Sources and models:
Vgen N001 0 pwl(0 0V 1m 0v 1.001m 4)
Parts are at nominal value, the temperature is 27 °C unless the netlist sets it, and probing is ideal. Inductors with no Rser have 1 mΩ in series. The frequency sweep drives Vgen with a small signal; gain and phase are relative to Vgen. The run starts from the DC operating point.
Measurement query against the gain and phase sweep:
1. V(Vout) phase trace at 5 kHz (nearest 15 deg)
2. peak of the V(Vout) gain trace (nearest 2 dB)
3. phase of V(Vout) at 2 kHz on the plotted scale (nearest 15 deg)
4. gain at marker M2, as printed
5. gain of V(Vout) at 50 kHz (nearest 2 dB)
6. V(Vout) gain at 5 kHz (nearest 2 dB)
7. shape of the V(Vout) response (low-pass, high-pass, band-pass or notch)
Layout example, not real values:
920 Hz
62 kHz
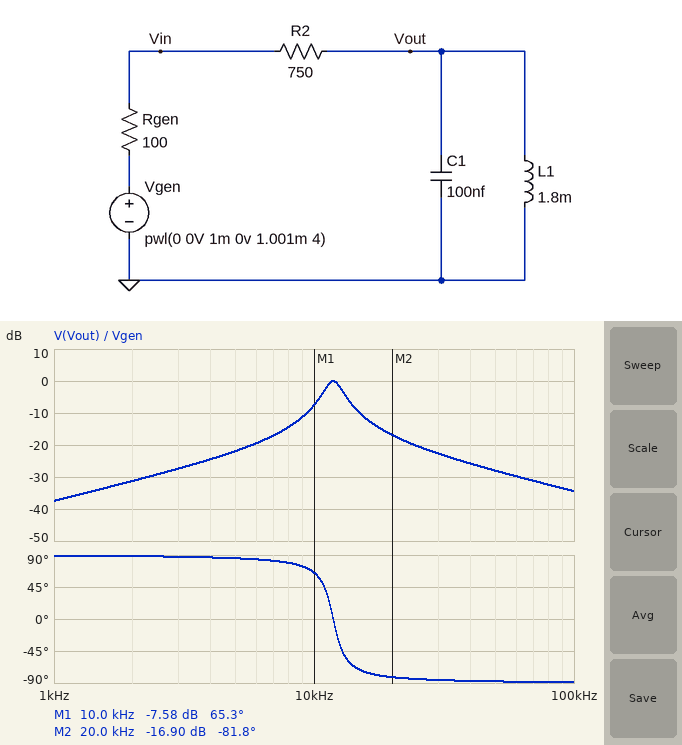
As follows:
90 deg
0 dB
90 deg
-16.90 dB
-28 dB
-22 dB
band-pass
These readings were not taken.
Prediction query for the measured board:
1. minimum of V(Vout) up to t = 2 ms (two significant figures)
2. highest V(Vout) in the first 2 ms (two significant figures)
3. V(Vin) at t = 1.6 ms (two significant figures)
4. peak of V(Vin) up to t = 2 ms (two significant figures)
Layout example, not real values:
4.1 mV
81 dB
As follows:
-440 mV
560 mV
3.5 V
3.6 V
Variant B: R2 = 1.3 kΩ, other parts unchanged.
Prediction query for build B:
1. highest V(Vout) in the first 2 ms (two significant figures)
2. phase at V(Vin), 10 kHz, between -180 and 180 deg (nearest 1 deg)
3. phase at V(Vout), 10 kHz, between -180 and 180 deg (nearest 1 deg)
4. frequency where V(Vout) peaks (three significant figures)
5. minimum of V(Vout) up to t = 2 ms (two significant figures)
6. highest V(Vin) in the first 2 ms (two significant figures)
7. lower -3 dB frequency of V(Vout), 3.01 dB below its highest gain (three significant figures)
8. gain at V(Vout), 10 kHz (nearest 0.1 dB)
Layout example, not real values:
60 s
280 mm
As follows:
360 mV
1 deg
74 deg
11.9 kHz
-310 mV
3.7 V
11.3 kHz
-11.4 dB
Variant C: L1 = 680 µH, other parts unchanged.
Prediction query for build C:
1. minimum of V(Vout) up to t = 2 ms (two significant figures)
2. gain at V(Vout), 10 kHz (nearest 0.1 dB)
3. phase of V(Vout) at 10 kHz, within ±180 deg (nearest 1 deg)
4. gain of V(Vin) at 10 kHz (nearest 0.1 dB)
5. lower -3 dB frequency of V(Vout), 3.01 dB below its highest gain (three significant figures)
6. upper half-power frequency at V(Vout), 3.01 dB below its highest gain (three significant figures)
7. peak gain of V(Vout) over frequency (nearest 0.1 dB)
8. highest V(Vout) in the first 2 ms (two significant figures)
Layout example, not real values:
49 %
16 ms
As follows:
-310 mV
-23.3 dB
86 deg
-1.1 dB
18.4 kHz
20.3 kHz
0 dB
360 mV
